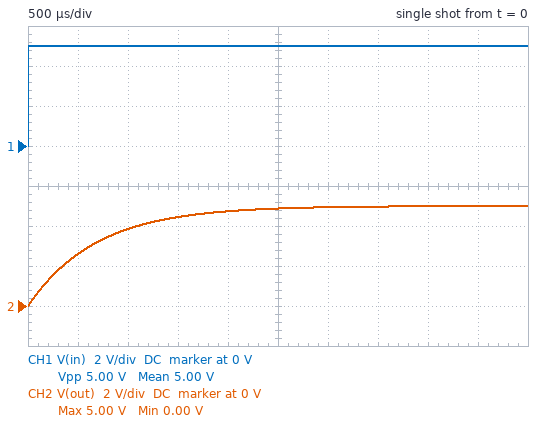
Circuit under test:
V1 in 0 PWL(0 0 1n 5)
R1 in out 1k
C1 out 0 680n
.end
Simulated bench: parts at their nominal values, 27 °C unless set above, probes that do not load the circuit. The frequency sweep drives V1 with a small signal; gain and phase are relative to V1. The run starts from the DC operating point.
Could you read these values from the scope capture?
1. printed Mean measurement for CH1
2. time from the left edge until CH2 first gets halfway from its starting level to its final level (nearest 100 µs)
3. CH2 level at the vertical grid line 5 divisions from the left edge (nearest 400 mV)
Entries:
5.00 V
500 µs
4.8 V
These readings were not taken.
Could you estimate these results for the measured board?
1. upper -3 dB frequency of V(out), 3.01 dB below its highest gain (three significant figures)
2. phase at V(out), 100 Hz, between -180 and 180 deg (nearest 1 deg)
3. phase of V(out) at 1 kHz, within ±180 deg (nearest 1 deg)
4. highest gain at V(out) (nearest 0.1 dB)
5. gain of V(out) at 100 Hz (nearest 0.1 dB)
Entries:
234 Hz
-23 deg
-77 deg
0 dB
-0.7 dB
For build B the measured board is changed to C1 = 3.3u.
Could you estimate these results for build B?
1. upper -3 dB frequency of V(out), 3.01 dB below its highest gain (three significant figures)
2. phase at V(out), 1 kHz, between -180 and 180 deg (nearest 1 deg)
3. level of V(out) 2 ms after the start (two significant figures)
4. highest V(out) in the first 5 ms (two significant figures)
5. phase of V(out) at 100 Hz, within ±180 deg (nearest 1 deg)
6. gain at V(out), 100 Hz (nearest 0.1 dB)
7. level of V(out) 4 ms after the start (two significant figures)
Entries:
48.2 Hz
-87 deg
2.3 V
3.9 V
-64 deg
-7.2 dB
3.5 V
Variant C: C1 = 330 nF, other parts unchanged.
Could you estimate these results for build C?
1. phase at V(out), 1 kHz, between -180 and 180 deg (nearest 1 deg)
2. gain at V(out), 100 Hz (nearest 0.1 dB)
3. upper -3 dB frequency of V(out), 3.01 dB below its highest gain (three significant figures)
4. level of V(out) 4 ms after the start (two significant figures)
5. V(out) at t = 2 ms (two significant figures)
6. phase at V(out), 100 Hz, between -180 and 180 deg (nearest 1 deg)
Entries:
-64 deg
-0.2 dB
482 Hz
5.0 V
5.0 V
-12 deg
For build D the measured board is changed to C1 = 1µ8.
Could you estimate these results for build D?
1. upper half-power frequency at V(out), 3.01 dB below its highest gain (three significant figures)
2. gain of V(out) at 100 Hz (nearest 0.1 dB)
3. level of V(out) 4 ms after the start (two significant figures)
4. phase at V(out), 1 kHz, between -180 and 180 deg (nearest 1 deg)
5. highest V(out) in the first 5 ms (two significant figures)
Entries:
88.4 Hz
-3.6 dB
4.5 V
-85 deg
4.7 V
